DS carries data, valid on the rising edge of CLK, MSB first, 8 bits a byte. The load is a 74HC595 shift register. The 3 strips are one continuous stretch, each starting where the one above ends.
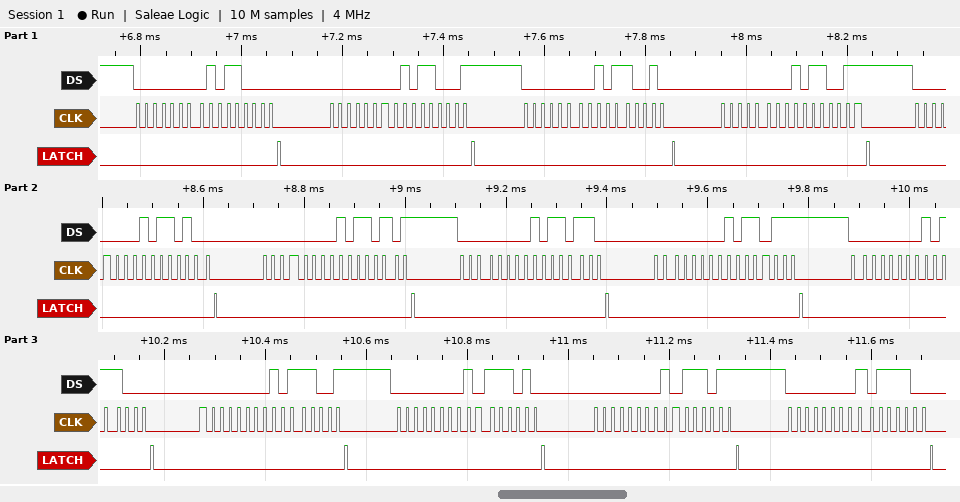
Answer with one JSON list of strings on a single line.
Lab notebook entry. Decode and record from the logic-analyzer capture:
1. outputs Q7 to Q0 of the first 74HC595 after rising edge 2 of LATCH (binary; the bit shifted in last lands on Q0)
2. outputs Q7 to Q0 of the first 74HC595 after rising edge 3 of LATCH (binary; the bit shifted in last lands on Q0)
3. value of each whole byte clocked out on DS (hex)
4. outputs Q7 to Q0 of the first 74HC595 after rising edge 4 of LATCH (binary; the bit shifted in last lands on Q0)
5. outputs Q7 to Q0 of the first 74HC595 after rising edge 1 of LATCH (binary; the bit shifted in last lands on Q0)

["10110001", "10110010", "00 B0 00 B1 00 B2 00 B3 00 B4 00 B5 00 B6 00 B7 00 B8 00 B9 00 BA 00 BB 00 BC", "10110011", "10110000"]
